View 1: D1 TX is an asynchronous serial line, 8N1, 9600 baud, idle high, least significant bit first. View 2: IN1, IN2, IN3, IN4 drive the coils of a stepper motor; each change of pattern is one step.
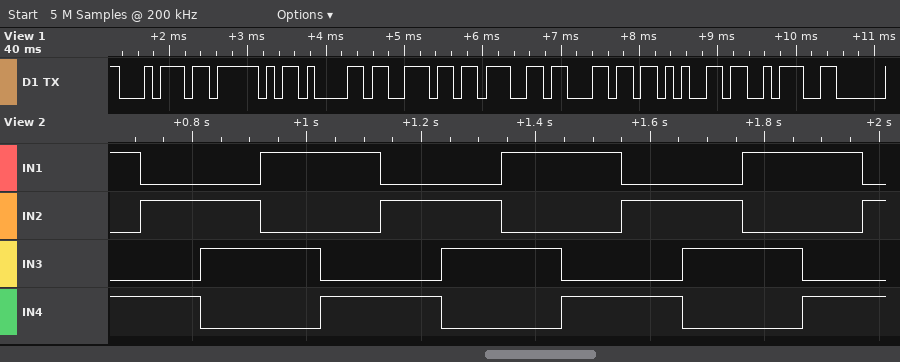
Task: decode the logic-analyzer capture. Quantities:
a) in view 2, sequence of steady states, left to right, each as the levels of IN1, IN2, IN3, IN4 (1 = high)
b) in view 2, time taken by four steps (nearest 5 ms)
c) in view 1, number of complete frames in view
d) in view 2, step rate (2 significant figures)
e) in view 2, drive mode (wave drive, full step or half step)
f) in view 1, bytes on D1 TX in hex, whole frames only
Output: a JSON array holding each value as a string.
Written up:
["1001 0101 0110 1010 1001 0101 0110 1010 1001 0101 0110 1010 1001 0101", "420 ms", "8", "9.5 steps/s", "full step", "0x74 0x5F 0x61 0x6E 0x67 0x6C 0x65 0x3A"]
